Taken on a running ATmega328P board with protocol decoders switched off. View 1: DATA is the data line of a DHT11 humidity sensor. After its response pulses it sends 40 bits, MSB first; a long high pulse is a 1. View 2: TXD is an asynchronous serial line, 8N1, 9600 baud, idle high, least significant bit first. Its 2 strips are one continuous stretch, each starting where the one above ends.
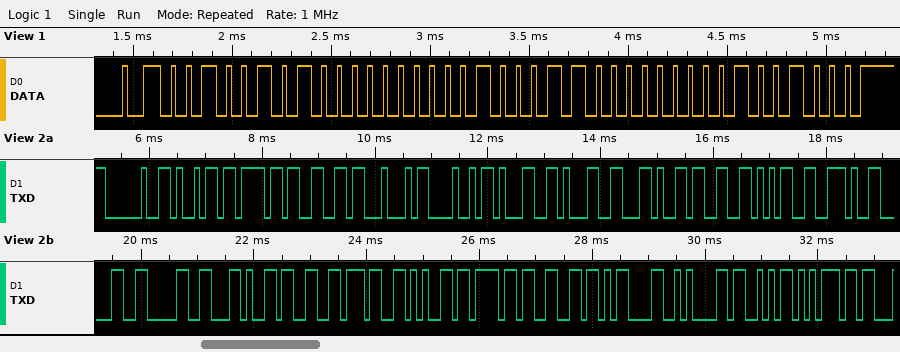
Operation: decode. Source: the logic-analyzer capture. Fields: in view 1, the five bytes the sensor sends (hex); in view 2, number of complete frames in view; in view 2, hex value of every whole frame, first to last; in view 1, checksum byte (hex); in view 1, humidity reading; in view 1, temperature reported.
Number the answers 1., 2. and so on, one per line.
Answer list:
1. 25 00 23 00 48
2. 24
3. 20 69 6F 66 44 48 31 31 2C 33 35 2E 30 30 2C 33 37 65 6F 66 0D 0A 53 75
4. 0x48
5. 37 %
6. 35.0 °C
